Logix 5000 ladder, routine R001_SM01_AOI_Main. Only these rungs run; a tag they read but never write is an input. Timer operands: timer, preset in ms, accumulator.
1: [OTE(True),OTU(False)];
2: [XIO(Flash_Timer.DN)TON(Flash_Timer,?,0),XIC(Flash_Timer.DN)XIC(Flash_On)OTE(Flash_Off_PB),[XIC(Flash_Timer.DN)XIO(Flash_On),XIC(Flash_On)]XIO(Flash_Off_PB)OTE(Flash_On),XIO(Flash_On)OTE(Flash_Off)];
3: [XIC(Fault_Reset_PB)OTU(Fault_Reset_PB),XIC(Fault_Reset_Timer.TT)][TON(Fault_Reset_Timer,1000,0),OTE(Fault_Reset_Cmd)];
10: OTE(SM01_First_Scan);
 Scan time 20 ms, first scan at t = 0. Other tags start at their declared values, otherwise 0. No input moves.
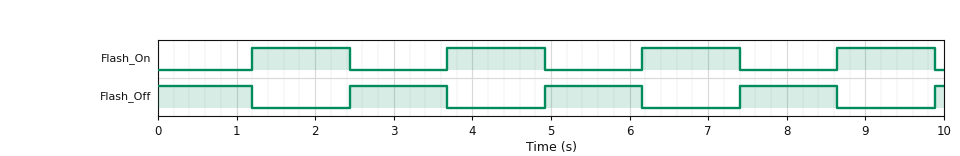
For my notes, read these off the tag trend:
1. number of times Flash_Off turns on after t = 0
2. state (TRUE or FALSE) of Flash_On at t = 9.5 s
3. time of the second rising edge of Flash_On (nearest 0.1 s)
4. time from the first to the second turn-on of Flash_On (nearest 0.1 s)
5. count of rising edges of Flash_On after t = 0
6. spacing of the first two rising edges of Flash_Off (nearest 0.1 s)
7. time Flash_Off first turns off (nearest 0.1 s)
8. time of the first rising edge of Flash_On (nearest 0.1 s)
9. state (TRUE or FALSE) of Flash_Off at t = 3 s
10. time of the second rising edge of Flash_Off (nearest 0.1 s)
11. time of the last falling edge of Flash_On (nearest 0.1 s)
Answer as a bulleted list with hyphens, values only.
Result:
- 4
- TRUE
- 3.7 s
- 2.5 s
- 4
- 2.5 s
- 1.2 s
- 1.2 s
- TRUE
- 4.9 s
- 9.9 s
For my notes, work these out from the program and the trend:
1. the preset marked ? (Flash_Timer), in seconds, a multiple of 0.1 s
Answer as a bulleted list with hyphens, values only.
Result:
- 1.2 s
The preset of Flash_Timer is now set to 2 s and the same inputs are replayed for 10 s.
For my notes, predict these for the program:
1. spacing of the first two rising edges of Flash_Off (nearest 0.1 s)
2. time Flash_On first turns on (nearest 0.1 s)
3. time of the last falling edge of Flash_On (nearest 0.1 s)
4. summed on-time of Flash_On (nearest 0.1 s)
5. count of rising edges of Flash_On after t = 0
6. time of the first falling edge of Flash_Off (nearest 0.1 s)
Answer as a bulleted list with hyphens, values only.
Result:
- 4.1 s
- 2.0 s
- 8.1 s
- 4.1 s
- 2
- 2.0 s
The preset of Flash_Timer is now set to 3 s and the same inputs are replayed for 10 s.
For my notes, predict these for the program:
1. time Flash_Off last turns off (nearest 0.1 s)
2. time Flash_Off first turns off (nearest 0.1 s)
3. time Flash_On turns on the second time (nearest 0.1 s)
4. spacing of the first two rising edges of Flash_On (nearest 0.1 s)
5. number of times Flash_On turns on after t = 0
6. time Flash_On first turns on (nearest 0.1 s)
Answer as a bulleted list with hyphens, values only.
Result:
- 9.1 s
- 3.0 s
- 9.1 s
- 6.1 s
- 2
- 3.0 s
